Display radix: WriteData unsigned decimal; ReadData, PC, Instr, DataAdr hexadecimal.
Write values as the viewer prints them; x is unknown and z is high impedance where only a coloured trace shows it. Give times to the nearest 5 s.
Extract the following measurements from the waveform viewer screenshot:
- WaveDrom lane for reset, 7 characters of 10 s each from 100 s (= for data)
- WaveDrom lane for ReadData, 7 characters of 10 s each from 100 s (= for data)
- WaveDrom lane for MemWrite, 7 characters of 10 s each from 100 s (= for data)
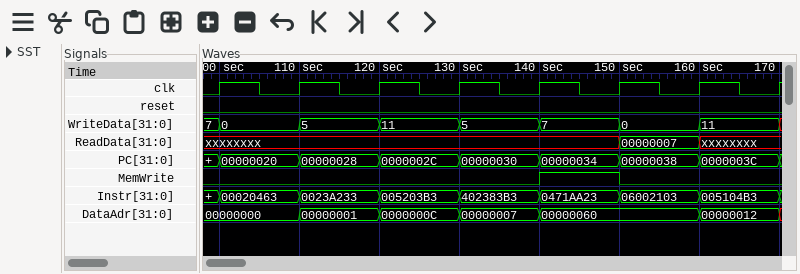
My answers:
{name: 'reset', wave: '0......'}
{name: 'ReadData', wave: 'x....=x', data: '00000007'}
{name: 'MemWrite', wave: '0...10.'}
